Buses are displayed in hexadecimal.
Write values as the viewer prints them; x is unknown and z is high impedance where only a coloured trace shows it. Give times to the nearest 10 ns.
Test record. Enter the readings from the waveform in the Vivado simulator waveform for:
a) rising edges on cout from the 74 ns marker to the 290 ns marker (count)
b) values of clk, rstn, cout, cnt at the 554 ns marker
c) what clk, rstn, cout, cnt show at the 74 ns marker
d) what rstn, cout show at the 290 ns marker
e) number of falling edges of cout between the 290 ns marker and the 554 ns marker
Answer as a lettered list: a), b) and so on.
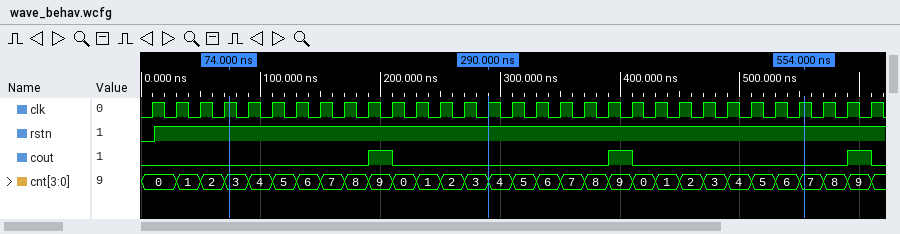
a) 1
b) clk=1, rstn=1, cout=0, cnt=7
c) clk=1, rstn=1, cout=0, cnt=3
d) rstn=1, cout=0
e) 1
